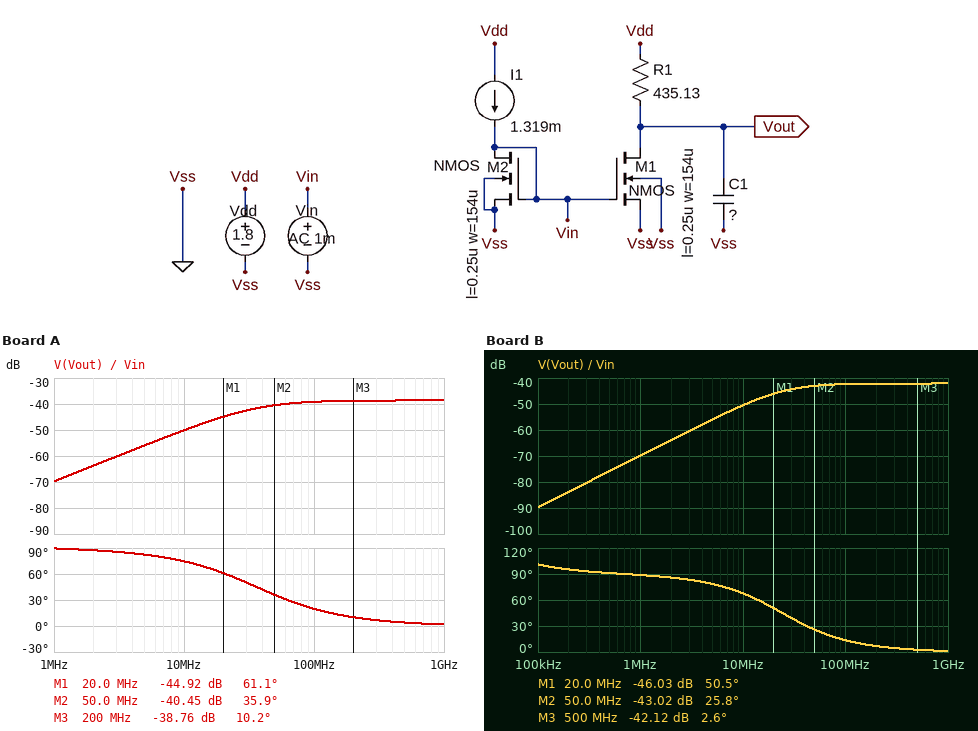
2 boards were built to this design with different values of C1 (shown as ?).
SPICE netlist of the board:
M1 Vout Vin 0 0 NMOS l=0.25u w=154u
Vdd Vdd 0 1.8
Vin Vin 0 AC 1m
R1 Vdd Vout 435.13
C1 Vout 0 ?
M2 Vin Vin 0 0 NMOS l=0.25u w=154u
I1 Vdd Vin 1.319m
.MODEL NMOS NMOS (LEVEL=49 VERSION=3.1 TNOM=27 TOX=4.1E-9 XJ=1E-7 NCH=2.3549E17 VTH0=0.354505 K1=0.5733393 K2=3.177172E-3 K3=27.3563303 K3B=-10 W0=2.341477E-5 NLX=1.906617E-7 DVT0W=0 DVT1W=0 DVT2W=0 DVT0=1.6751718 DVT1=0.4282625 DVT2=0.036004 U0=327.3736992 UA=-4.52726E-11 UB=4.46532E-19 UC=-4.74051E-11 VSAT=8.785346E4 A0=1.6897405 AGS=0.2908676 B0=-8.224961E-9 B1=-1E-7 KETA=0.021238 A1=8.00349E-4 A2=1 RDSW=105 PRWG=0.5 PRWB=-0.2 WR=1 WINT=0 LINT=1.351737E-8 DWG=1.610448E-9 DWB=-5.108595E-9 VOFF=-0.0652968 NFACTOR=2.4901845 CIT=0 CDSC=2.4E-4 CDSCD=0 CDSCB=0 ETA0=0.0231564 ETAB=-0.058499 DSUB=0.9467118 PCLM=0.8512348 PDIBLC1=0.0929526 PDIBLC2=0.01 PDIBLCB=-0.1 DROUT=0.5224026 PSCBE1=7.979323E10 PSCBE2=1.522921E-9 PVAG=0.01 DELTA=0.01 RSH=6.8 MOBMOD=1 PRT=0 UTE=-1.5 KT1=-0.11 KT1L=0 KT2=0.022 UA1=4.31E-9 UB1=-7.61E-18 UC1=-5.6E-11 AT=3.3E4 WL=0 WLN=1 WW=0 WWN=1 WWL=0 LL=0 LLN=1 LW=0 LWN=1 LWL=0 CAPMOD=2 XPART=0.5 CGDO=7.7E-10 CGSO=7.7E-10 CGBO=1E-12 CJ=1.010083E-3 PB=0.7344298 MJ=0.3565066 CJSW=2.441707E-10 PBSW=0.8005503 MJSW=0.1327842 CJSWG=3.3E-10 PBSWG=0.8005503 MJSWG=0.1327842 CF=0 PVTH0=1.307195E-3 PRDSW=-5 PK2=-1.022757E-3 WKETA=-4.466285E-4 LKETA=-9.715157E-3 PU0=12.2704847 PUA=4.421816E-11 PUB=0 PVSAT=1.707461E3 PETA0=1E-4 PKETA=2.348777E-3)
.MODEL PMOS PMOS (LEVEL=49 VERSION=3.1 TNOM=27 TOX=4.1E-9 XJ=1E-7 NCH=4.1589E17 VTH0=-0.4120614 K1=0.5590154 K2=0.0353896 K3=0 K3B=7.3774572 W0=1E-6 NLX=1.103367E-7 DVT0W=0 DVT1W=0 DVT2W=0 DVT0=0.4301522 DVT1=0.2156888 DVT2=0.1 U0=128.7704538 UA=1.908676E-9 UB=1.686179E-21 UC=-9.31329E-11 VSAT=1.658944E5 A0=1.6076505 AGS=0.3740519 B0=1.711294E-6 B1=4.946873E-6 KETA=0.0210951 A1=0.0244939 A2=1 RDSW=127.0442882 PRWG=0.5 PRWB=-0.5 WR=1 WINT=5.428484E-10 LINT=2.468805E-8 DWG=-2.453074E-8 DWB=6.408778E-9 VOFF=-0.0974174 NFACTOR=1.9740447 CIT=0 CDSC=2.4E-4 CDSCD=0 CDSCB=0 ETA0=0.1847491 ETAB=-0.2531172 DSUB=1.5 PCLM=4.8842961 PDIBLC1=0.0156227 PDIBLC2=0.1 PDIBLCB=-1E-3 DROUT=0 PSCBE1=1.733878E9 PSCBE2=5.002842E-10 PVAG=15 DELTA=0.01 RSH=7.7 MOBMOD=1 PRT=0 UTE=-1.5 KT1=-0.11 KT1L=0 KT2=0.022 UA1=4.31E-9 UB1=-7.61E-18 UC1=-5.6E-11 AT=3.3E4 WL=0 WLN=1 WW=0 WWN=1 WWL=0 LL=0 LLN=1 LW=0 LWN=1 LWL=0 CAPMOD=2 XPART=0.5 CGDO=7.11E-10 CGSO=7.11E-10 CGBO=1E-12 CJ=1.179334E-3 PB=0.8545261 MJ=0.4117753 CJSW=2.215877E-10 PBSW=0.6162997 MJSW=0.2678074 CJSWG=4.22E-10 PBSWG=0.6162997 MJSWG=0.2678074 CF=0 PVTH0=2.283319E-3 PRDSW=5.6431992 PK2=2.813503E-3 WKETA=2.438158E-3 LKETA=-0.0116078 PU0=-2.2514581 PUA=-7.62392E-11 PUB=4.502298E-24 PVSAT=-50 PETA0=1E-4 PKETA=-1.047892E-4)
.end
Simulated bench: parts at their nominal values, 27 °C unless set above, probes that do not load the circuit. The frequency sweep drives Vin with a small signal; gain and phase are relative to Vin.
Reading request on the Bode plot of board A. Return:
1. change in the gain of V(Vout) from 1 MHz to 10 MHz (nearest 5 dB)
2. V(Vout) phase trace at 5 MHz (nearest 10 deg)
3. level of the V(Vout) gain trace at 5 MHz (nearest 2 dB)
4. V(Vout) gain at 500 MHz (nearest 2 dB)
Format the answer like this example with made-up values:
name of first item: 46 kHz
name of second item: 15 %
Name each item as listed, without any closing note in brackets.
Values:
change in the gain of V(Vout) from 1 MHz to 10 MHz: 20 dB
V(Vout) phase trace at 5 MHz: 80 deg
level of the V(Vout) gain trace at 5 MHz: -56 dB
V(Vout) gain at 500 MHz: -38 dB
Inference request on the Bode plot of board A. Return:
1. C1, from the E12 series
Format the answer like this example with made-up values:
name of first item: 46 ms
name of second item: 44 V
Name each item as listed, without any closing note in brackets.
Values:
C1, from the E12 series: 10 pF
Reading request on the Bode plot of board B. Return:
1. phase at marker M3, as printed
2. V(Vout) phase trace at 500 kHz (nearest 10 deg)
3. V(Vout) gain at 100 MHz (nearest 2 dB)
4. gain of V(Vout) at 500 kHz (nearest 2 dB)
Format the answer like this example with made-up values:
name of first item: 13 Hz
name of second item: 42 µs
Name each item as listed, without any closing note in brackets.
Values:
phase at marker M3, as printed: 2.6 deg
V(Vout) phase trace at 500 kHz: 90 deg
V(Vout) gain at 100 MHz: -42 dB
gain of V(Vout) at 500 kHz: -76 dB
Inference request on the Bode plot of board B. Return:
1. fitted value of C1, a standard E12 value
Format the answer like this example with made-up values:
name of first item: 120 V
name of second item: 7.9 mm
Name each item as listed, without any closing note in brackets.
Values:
fitted value of C1, a standard E12 value: 15 pF
